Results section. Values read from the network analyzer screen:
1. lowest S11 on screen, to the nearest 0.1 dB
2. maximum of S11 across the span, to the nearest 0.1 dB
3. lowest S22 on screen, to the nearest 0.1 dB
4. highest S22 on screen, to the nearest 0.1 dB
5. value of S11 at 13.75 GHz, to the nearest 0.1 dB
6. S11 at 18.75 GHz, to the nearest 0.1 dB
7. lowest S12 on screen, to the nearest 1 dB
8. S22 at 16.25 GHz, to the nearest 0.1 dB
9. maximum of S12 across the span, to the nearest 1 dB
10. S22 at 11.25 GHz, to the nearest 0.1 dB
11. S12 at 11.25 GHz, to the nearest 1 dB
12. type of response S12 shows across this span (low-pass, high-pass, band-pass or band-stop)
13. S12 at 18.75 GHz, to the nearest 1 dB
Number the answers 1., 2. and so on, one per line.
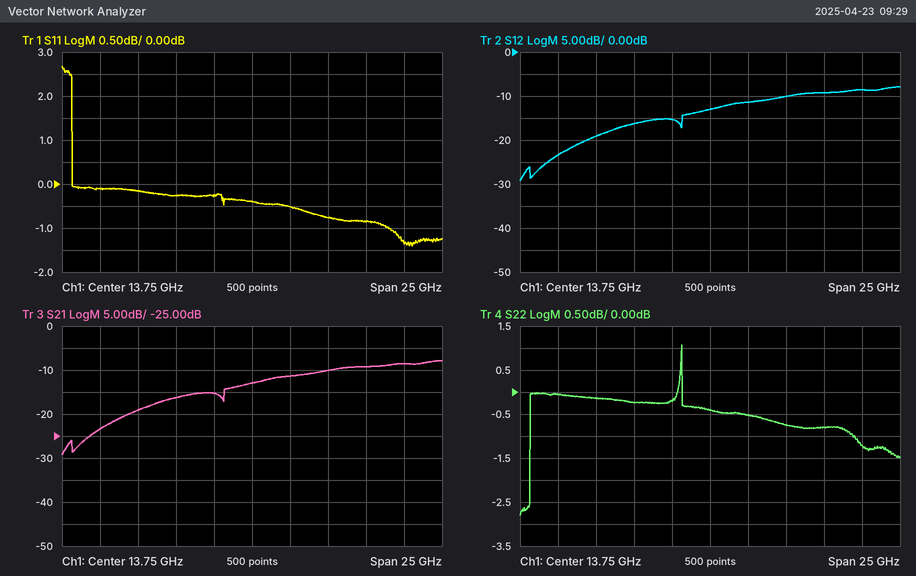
1. -1.4 dB
2. 2.7 dB
3. -2.8 dB
4. 1.1 dB
5. -0.4 dB
6. -0.8 dB
7. -29 dB
8. -0.5 dB
9. -8 dB
10. -0.2 dB
11. -15 dB
12. high-pass
13. -10 dB
